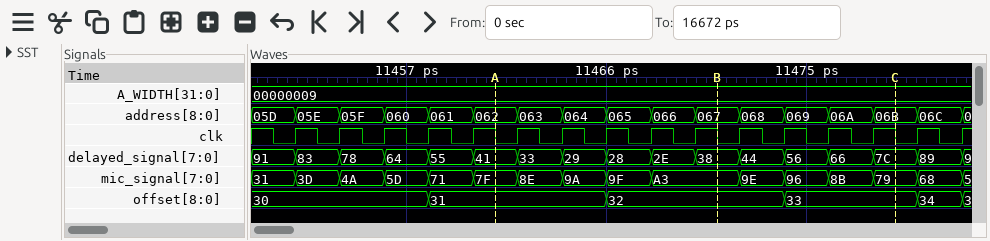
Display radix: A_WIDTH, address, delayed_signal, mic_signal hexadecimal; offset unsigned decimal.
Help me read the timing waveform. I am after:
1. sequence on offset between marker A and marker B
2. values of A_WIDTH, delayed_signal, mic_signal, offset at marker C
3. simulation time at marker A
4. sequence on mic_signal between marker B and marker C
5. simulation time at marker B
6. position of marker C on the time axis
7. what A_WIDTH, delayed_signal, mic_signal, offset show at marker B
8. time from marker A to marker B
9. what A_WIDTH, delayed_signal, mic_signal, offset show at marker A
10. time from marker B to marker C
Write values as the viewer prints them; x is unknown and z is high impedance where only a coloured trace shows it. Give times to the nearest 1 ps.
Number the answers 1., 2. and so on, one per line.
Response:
1. 31, 32
2. A_WIDTH=00000009, delayed_signal=7C, mic_signal=79, offset=33
3. 11461 ps
4. A3, 9E, 96, 8B, 79
5. 11471 ps
6. 11479 ps
7. A_WIDTH=00000009, delayed_signal=38, mic_signal=A3, offset=32
8. 10 ps
9. A_WIDTH=00000009, delayed_signal=41, mic_signal=7F, offset=31
10. 8 ps
